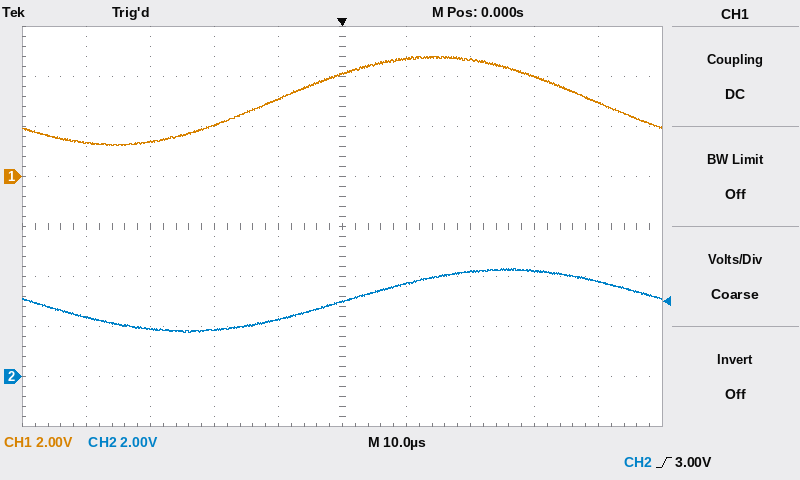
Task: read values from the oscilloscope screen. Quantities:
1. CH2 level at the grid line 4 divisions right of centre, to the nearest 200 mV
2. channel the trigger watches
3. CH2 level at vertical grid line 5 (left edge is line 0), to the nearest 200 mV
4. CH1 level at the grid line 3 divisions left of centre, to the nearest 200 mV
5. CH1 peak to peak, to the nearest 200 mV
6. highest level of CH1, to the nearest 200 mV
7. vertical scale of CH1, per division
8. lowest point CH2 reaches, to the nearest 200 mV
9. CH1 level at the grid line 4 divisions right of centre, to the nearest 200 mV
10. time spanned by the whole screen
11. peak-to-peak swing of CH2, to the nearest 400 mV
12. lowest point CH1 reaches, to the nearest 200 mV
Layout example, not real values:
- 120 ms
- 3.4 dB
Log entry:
- 3.8 V
- CH2
- 3.0 V
- 1.4 V
- 3.6 V
- 4.8 V
- 2 V
- 1.8 V
- 3.0 V
- 100 µs
- 2.4 V
- 1.2 V
